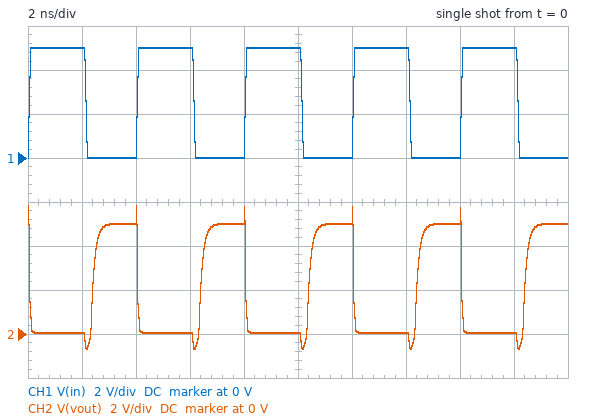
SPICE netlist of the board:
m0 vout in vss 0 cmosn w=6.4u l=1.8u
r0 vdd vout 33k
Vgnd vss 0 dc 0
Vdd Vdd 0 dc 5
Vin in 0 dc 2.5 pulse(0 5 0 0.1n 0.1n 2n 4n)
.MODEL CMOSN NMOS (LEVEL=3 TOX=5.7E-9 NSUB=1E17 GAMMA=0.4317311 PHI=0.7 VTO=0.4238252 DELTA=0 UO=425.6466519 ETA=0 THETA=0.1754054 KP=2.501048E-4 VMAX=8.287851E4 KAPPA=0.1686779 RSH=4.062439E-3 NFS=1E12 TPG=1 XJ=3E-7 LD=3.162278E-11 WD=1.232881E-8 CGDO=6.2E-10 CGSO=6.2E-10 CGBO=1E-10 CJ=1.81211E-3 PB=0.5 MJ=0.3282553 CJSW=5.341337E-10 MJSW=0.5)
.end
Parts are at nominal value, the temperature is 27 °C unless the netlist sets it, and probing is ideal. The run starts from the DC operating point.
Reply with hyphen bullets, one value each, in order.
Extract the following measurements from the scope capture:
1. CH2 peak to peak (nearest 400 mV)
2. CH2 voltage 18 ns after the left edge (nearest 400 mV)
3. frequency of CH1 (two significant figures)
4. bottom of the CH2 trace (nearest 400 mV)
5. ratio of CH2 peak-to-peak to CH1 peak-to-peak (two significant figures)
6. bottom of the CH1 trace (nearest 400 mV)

- 6.4 V
- 0 V
- 250 MHz
- -800 mV
- 1.3
- 0 V
